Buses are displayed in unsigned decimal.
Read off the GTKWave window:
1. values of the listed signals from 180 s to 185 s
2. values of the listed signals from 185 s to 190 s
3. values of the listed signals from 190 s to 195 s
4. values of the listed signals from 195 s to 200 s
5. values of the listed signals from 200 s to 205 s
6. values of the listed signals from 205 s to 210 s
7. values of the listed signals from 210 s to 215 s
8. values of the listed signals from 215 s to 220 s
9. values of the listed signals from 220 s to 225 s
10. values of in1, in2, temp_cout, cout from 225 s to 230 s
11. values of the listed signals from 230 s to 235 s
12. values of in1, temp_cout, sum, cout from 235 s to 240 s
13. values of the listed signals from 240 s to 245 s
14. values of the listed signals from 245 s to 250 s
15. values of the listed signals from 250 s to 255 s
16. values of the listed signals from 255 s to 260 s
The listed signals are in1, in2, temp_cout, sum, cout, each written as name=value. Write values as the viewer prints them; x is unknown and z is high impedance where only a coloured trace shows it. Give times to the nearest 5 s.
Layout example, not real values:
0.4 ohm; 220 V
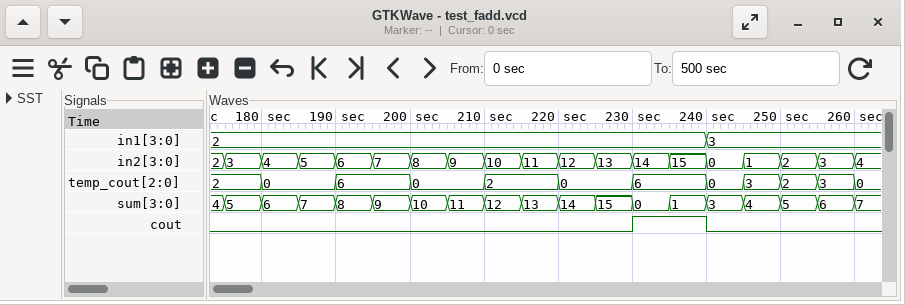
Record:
in1=2, in2=4, temp_cout=0, sum=6, cout=0; in1=2, in2=5, temp_cout=0, sum=7, cout=0; in1=2, in2=6, temp_cout=6, sum=8, cout=0; in1=2, in2=7, temp_cout=6, sum=9, cout=0; in1=2, in2=8, temp_cout=0, sum=10, cout=0; in1=2, in2=9, temp_cout=0, sum=11, cout=0; in1=2, in2=10, temp_cout=2, sum=12, cout=0; in1=2, in2=11, temp_cout=2, sum=13, cout=0; in1=2, in2=12, temp_cout=0, sum=14, cout=0; in1=2, in2=13, temp_cout=0, cout=0; in1=2, in2=14, temp_cout=6, sum=0, cout=1; in1=2, temp_cout=6, sum=1, cout=1; in1=3, in2=0, temp_cout=0, sum=3, cout=0; in1=3, in2=1, temp_cout=3, sum=4, cout=0; in1=3, in2=2, temp_cout=2, sum=5, cout=0; in1=3, in2=3, temp_cout=3, sum=6, cout=0
